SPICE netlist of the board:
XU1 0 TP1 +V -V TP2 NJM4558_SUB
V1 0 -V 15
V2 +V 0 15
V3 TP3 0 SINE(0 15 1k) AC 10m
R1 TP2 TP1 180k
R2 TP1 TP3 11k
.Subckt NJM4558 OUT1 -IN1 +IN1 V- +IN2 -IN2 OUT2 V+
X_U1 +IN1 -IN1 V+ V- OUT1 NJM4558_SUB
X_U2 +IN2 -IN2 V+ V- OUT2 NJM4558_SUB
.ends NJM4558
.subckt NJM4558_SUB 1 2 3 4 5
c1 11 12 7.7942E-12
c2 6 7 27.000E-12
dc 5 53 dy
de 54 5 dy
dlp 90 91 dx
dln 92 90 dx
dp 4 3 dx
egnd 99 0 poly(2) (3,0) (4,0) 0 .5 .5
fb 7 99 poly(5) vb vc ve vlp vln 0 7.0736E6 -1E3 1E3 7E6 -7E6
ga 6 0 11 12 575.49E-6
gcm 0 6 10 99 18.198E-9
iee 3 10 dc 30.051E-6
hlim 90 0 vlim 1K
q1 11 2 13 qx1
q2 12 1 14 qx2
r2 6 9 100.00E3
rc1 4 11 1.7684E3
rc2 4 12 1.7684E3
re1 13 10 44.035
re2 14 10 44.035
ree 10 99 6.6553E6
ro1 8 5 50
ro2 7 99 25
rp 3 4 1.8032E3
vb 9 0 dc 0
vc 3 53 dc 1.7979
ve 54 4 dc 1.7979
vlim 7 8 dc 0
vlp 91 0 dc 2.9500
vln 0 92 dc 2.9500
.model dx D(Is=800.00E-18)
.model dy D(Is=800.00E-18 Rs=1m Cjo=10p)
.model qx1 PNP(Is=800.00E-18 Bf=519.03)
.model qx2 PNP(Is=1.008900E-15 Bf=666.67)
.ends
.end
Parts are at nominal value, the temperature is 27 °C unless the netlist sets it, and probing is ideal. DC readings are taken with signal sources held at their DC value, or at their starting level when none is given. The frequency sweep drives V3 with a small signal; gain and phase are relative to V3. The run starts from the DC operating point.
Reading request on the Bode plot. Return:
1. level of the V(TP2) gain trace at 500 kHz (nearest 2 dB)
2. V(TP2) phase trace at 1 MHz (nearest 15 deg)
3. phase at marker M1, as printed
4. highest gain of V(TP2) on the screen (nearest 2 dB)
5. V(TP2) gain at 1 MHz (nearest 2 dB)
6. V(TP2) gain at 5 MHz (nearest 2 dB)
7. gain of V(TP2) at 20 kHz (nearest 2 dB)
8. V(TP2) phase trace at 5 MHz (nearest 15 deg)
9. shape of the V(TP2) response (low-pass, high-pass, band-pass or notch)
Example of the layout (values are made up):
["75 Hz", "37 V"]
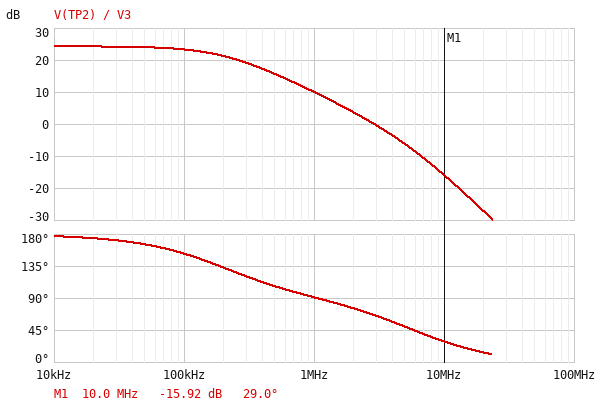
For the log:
["16 dB", "90 deg", "29.0 deg", "24 dB", "10 dB", "-6 dB", "24 dB", "45 deg", "low-pass"]
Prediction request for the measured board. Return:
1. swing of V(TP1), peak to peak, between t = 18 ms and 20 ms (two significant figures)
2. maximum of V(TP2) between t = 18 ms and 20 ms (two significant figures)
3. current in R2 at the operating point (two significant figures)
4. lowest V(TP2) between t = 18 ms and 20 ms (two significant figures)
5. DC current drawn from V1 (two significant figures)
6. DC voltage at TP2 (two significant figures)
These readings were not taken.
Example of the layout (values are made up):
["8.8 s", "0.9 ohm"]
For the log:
["27 V", "14 V", "550 nA", "-14 V", "17 mA", "-110 mV"]
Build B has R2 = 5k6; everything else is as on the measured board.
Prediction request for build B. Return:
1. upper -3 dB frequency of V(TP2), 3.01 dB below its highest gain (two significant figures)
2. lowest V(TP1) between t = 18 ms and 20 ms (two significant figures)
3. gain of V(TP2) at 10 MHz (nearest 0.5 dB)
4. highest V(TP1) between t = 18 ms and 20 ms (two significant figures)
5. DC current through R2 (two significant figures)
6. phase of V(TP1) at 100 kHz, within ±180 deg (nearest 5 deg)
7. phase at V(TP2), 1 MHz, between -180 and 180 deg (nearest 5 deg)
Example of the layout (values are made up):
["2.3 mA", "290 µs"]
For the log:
["100 kHz", "-14 V", "-15.5 dB", "14 V", "1.1 µA", "45 deg", "85 deg"]
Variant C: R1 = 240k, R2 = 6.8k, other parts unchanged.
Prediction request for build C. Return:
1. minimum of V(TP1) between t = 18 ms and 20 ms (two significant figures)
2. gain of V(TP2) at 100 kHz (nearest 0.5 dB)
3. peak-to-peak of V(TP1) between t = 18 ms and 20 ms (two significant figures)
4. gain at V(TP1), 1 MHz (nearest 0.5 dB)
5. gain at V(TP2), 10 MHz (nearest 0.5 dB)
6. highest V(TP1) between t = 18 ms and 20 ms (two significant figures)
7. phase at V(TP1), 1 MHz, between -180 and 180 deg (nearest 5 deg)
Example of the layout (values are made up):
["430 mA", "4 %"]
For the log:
["-14 V", "27.5 dB", "28 V", "0 dB", "-15.5 dB", "14 V", "5 deg"]
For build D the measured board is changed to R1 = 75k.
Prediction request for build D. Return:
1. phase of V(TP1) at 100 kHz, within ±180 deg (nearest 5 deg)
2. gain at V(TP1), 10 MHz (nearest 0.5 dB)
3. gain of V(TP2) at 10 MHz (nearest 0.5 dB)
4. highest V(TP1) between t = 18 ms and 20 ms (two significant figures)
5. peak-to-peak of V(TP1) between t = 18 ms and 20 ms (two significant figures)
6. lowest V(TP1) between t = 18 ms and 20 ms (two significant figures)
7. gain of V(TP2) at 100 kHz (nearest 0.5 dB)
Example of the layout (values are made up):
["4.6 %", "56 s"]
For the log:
["80 deg", "-1.0 dB", "-16.5 dB", "11 V", "23 V", "-11 V", "16.5 dB"]
